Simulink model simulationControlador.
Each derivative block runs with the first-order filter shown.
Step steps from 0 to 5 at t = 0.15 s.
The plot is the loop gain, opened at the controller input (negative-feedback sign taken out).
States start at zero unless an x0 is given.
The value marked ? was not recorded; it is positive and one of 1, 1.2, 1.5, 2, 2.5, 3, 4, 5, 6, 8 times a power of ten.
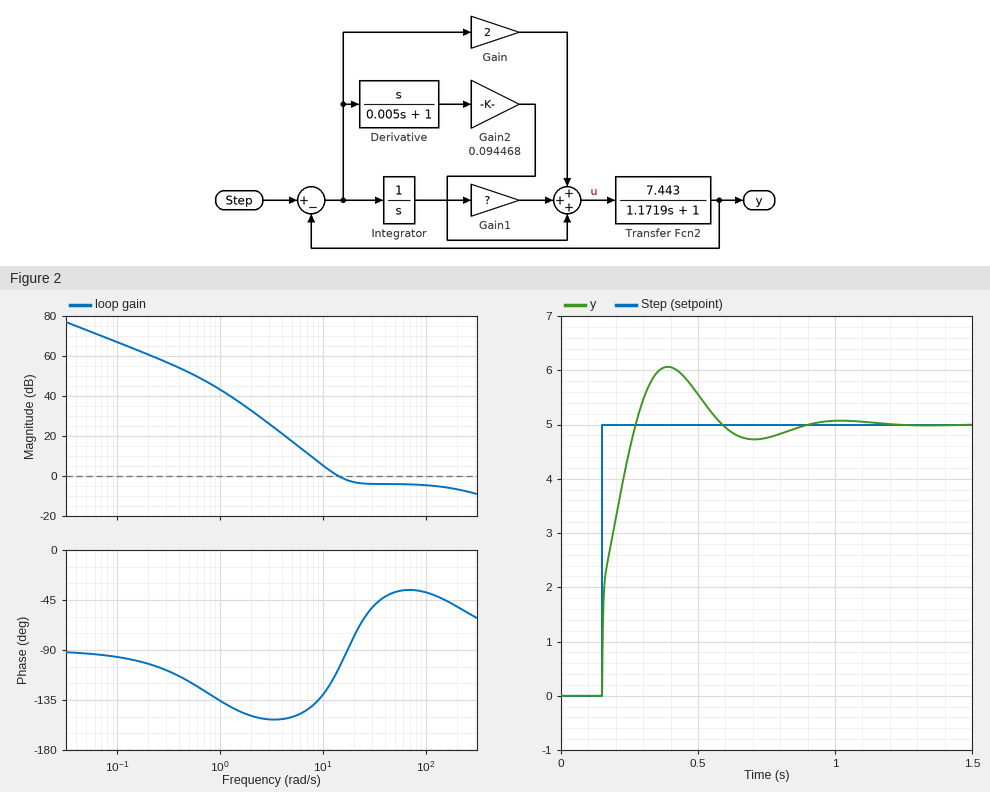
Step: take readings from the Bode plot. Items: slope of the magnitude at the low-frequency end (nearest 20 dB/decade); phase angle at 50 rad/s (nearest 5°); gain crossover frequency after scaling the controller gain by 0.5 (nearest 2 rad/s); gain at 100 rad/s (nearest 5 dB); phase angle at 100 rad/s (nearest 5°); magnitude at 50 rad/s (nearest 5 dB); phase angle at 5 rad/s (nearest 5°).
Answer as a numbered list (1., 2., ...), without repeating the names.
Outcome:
1. -20 dB/decade
2. -40°
3. 10 rad/s
4. -5 dB
5. -40°
6. -5 dB
7. -150°
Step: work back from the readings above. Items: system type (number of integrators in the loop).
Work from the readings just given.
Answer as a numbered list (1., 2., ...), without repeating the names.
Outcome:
1. 1
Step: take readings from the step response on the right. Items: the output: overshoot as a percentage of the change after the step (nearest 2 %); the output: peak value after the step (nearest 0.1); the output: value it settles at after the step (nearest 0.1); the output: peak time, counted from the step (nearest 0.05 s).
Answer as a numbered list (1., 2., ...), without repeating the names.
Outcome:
1. 22 %
2. 6.1
3. 5.0
4. 0.25 s
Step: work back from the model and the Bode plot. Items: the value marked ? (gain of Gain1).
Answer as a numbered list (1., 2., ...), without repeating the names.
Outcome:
1. 30
